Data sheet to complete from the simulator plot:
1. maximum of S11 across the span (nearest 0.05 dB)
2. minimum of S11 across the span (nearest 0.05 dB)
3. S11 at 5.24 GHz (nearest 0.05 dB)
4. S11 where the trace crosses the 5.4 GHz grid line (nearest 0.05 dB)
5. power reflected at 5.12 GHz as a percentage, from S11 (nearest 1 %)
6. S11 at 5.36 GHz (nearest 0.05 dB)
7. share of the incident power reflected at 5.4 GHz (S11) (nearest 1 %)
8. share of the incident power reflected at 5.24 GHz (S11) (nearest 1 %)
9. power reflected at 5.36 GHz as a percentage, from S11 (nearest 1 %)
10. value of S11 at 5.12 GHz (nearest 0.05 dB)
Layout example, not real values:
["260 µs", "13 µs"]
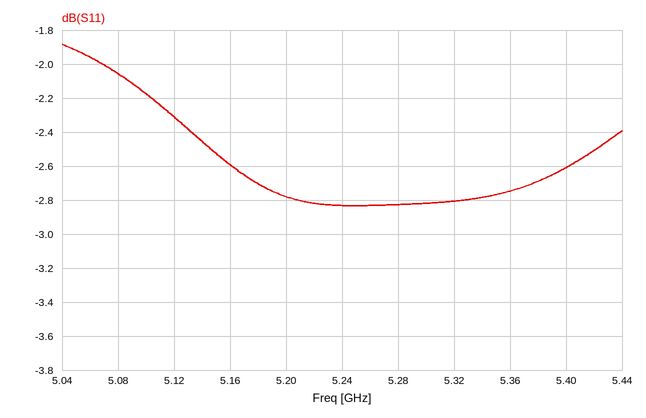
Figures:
["-1.90 dB", "-2.85 dB", "-2.85 dB", "-2.60 dB", "59 %", "-2.75 dB", "55 %", "52 %", "53 %", "-2.30 dB"]
